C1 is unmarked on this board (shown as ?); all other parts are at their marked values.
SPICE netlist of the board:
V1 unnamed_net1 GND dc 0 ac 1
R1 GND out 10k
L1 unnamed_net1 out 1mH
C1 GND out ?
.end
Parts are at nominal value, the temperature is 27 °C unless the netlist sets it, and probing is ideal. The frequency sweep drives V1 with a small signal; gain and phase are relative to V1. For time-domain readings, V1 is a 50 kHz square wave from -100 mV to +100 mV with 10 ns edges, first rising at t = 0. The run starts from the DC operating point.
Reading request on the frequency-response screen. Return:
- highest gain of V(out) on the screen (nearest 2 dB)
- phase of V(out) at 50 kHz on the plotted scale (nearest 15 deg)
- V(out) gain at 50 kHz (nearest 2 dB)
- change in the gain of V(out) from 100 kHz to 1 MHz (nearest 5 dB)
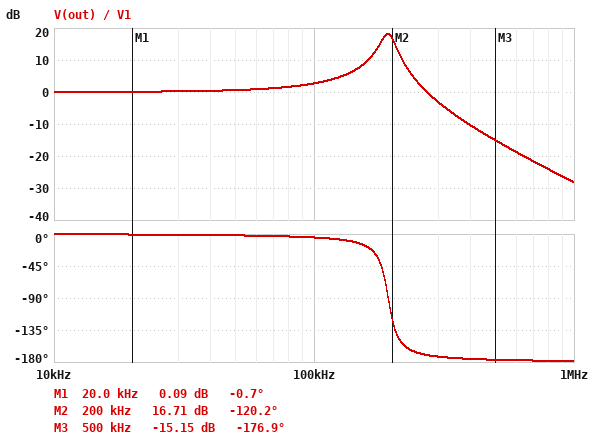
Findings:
18 dB
0 deg
0 dB
-30 dB
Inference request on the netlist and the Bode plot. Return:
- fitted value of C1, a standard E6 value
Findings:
680 pF
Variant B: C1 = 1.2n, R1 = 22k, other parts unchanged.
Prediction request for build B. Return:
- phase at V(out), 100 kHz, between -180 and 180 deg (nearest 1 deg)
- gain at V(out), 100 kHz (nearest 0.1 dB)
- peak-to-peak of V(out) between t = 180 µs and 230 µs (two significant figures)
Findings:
-3 deg
5.6 dB
1.3 V
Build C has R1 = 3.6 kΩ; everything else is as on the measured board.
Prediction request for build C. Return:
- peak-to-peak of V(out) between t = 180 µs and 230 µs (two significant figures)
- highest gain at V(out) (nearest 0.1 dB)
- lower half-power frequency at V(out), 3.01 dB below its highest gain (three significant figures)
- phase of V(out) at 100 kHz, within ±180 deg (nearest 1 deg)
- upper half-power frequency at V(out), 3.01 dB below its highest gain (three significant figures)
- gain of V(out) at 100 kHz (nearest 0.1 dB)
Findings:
410 mV
9.6 dB
151 kHz
-13 deg
218 kHz
2.5 dB
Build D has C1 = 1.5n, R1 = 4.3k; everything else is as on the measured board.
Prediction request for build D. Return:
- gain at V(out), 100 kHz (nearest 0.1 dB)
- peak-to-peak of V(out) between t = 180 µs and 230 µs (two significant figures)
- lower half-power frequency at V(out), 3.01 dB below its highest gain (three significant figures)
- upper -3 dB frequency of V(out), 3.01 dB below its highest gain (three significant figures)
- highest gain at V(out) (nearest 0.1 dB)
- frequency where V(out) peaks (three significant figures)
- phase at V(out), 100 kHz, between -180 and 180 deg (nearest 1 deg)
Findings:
7.3 dB
490 mV
116 kHz
141 kHz
14.5 dB
129 kHz
-20 deg
